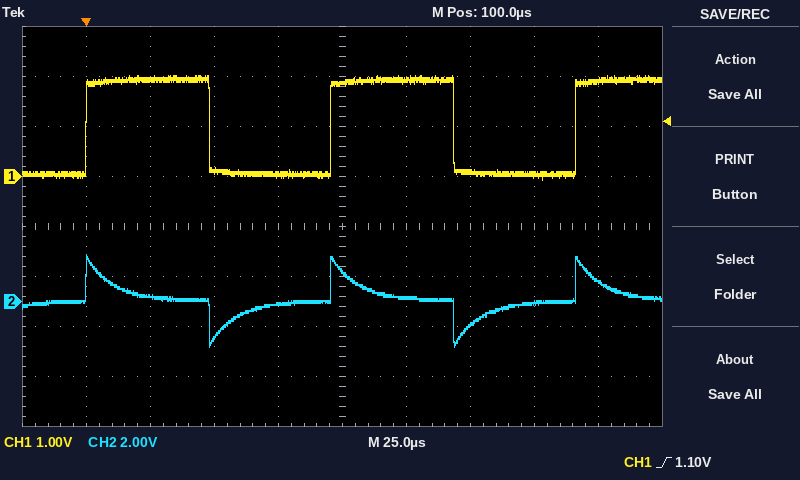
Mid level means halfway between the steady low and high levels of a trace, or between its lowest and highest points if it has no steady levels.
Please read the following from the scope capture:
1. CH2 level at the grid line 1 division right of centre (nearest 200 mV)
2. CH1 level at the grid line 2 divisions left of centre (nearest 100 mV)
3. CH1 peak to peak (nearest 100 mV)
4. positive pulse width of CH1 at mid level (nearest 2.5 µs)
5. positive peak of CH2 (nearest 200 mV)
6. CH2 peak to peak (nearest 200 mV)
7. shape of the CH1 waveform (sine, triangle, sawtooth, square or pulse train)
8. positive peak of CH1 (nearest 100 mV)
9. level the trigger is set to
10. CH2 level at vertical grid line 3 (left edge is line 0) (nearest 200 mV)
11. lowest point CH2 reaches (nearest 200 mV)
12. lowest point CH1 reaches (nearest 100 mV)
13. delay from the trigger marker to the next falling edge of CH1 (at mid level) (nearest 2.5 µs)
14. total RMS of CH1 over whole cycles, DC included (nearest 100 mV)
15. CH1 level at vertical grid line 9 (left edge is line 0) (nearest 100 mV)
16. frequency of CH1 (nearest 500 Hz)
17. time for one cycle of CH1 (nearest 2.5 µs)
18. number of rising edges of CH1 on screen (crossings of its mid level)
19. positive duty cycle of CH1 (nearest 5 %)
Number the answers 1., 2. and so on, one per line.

1. 200 mV
2. 100 mV
3. 2.1 V
4. 47.5 µs
5. 1.8 V
6. 3.6 V
7. square
8. 2.0 V
9. 1.10 V
10. -1.4 V
11. -1.8 V
12. -100 mV
13. 47.5 µs
14. 1.4 V
15. 1.9 V
16. 10.5 kHz
17. 95.0 µs
18. 3
19. 50 %
